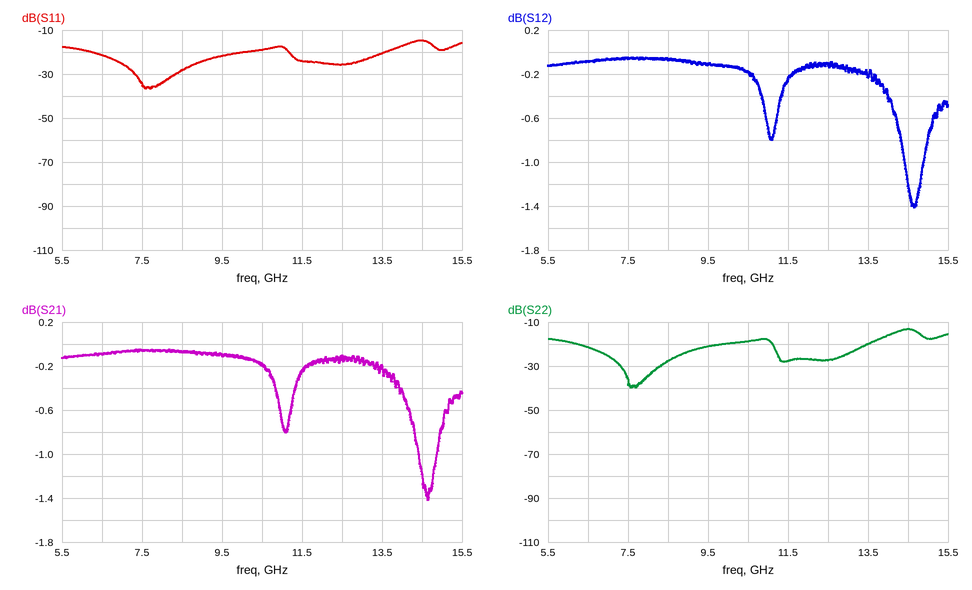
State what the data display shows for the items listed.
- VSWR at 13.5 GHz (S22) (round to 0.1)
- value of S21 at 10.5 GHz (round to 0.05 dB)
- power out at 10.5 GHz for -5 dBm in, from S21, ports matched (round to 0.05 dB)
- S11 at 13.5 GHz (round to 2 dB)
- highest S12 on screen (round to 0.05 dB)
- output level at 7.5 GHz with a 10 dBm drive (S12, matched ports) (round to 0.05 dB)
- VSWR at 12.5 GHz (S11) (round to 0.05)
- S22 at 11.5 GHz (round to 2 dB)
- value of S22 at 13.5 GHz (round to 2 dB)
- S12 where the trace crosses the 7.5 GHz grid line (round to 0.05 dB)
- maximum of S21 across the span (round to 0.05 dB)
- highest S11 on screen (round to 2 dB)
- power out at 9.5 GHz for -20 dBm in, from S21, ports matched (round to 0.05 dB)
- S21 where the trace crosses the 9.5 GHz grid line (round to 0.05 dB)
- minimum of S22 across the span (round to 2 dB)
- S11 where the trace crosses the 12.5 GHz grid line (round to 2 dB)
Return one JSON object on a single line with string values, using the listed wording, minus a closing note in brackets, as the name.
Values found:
{"VSWR at 13.5 GHz (S22)": "1.2", "value of S21 at 10.5 GHz": "-0.20 dB", "power out at 10.5 GHz for -5 dBm in, from S21, ports matched": "-5.20 dBm", "S11 at 13.5 GHz": "-20 dB", "highest S12 on screen": "-0.05 dB", "output level at 7.5 GHz with a 10 dBm drive (S12, matched ports)": "9.95 dBm", "VSWR at 12.5 GHz (S11)": "1.10", "S22 at 11.5 GHz": "-28 dB", "value of S22 at 13.5 GHz": "-20 dB", "S12 where the trace crosses the 7.5 GHz grid line": "-0.05 dB", "maximum of S21 across the span": "-0.05 dB", "highest S11 on screen": "-14 dB", "power out at 9.5 GHz for -20 dBm in, from S21, ports matched": "-20.10 dBm", "S21 where the trace crosses the 9.5 GHz grid line": "-0.10 dB", "minimum of S22 across the span": "-40 dB", "S11 where the trace crosses the 12.5 GHz grid line": "-26 dB"}
